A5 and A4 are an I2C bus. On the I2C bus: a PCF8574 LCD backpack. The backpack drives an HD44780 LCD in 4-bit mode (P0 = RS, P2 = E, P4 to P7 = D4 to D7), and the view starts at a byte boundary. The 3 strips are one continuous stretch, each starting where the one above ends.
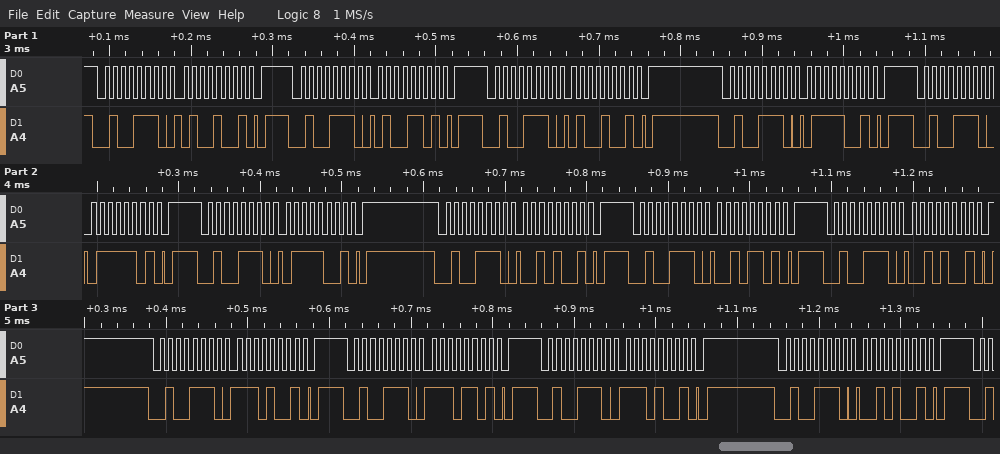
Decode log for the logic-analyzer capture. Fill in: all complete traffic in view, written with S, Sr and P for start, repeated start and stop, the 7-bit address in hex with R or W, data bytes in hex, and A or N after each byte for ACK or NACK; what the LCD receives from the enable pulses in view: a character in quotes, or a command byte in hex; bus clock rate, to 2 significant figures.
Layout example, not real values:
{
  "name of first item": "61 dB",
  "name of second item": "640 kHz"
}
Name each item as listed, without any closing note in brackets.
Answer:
{
  "all complete traffic in view, written with S, Sr and P for start, repeated start and stop, the 7-bit address in hex with R or W, data bytes in hex, and A or N after each byte for ACK or NACK": "S 27W A 49 A P S 27W A 4D A P S 27W A 49 A P S 27W A 79 A P S 27W A 7D A P S 27W A 79 A P S 27W A 29 A P S 27W A 2D A P S 27W A 29 A P S 27W A E9 A P S 27W A ED A P S 27W A E9 A P S 27W A 29 A P",
  "what the LCD receives from the enable pulses in view: a character in quotes, or a command byte in hex": "'G' '.'",
  "bus clock rate, to 2 significant figures": "100 kHz"
}
